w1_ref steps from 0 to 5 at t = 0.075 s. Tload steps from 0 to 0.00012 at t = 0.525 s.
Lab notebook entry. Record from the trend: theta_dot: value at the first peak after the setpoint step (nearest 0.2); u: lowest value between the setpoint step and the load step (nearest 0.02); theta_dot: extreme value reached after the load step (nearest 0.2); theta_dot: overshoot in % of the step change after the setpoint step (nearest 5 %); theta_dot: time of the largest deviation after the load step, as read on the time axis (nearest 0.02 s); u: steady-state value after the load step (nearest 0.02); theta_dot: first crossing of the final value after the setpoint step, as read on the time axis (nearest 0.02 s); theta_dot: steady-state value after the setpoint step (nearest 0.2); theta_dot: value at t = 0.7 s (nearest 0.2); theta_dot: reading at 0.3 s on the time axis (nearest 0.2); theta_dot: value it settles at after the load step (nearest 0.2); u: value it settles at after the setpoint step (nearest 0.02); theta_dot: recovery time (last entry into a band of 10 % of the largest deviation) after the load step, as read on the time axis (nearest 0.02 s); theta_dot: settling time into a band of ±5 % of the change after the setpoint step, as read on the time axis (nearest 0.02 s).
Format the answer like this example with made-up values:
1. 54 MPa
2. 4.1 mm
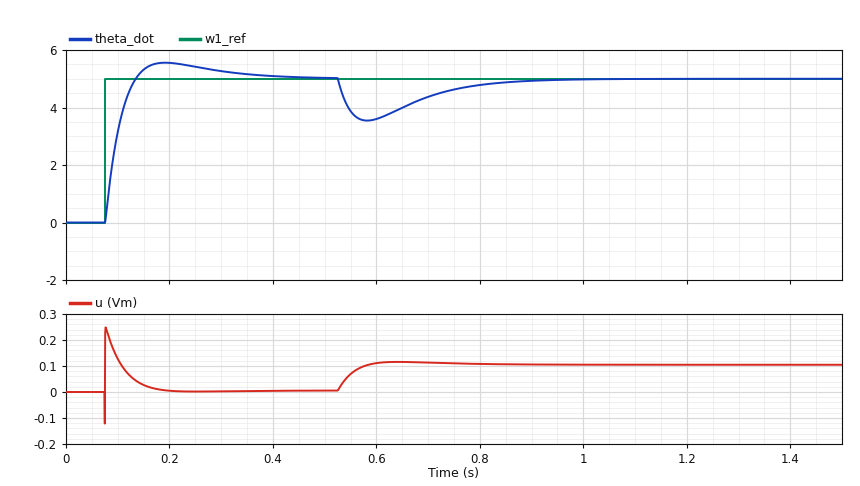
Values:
1. 5.6
2. -0.12
3. 3.6
4. 10 %
5. 0.58 s
6. 0.10
7. 0.14 s
8. 5.0
9. 4.4
10. 5.2
11. 5.0
12. 0.00
13. 0.84 s
14. 0.30 s
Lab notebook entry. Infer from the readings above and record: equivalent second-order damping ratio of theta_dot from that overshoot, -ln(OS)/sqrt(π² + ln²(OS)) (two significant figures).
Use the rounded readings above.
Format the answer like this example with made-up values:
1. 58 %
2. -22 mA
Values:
1. 0.59
